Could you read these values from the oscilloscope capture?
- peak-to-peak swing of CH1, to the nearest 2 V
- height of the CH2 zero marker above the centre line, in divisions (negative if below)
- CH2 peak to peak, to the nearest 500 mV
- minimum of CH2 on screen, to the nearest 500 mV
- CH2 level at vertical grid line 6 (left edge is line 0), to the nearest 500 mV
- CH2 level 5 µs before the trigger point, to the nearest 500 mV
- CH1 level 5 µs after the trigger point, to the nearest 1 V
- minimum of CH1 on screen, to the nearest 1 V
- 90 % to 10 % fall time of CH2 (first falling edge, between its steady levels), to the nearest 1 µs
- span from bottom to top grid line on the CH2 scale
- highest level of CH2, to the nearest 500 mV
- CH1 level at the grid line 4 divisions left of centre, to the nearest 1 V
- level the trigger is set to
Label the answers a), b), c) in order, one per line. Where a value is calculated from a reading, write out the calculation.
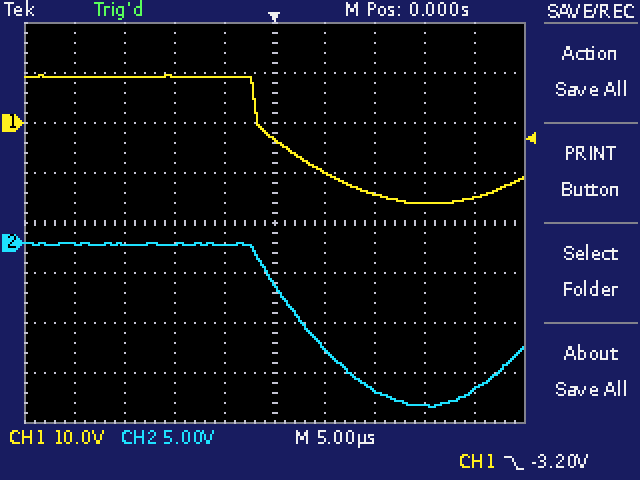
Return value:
a) 26 V
b) -0.4 div
c) 0.0 V − (-16.5 V) = 16.5 V
d) -16.5 V
e) -10.5 V
f) 0.0 V
g) -10 V
h) -16 V
i) 11 µs
j) 40 V
k) 0.0 V
l) 9 V
m) -3.20 V
